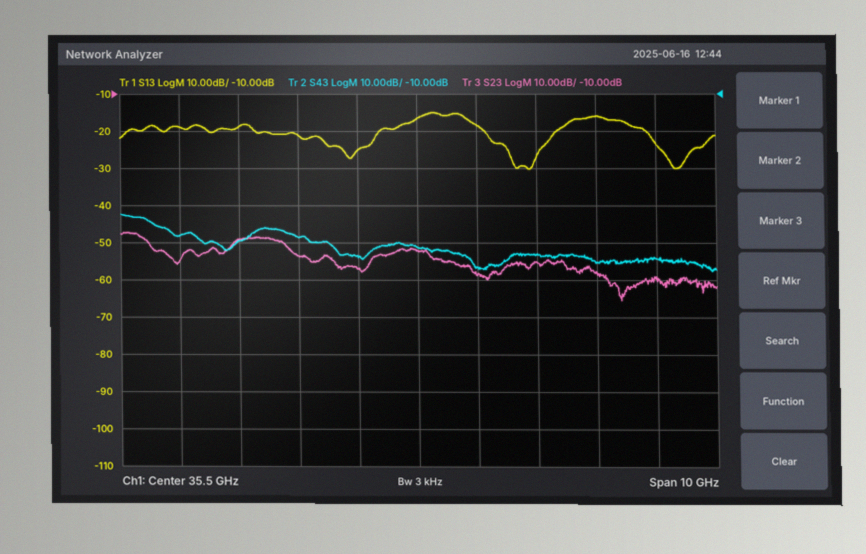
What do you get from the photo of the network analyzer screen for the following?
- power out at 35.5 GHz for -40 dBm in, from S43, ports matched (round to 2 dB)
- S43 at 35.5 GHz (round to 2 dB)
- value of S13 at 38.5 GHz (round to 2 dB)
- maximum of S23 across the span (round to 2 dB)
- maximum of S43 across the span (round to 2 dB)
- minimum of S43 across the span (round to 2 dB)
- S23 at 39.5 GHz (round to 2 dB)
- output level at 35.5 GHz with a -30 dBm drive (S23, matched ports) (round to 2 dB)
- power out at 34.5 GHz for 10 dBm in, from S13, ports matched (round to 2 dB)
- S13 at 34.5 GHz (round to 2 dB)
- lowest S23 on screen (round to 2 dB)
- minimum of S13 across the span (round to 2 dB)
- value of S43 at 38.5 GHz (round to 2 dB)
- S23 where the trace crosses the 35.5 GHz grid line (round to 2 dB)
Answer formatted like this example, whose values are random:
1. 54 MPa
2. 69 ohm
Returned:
1. -92 dBm
2. -52 dB
3. -16 dB
4. -48 dB
5. -42 dB
6. -58 dB
7. -60 dB
8. -82 dBm
9. -16 dBm
10. -26 dB
11. -66 dB
12. -30 dB
13. -56 dB
14. -52 dB
